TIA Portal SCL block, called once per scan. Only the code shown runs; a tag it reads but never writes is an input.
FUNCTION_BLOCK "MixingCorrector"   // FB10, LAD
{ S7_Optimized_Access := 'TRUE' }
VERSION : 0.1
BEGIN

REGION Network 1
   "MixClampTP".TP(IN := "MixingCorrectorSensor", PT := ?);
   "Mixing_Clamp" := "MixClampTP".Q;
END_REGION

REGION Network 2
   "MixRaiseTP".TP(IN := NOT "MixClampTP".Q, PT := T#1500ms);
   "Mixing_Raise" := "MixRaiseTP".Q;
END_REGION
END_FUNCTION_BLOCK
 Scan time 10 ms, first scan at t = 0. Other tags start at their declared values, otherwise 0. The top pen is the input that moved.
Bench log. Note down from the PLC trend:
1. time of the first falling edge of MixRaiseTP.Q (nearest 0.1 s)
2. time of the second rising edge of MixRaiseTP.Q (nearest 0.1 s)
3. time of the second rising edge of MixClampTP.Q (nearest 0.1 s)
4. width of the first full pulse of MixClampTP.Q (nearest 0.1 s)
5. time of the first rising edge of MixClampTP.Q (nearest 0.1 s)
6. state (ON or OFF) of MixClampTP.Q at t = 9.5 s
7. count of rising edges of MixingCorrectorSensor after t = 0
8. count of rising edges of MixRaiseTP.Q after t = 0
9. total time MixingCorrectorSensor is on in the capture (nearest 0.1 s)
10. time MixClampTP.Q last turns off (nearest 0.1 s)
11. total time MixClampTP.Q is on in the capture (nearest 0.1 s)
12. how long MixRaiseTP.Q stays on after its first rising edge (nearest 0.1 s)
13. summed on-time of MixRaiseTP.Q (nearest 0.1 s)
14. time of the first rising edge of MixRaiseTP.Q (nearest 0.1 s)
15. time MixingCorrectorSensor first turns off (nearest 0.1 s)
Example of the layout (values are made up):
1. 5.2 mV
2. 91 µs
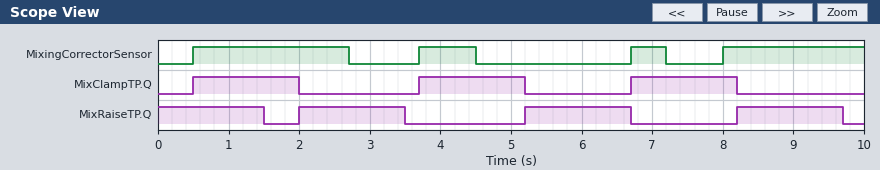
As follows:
1. 1.5 s
2. 5.2 s
3. 3.7 s
4. 1.5 s
5. 0.5 s
6. OFF
7. 4
8. 3
9. 5.5 s
10. 8.2 s
11. 4.5 s
12. 1.5 s
13. 6.0 s
14. 2.0 s
15. 2.7 s
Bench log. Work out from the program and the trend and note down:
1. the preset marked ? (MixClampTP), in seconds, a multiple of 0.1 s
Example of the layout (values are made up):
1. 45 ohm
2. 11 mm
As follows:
1. 1.5 s
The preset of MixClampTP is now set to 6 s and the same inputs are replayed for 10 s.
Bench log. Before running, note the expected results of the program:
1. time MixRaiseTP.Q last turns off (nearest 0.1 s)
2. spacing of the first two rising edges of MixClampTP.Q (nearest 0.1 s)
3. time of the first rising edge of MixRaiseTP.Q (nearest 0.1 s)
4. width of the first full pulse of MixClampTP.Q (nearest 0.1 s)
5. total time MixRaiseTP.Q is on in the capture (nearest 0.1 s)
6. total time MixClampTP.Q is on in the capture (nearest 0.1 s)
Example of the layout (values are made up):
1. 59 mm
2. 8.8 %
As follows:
1. 8.0 s
2. 6.2 s
3. 6.5 s
4. 6.0 s
5. 3.0 s
6. 9.3 s
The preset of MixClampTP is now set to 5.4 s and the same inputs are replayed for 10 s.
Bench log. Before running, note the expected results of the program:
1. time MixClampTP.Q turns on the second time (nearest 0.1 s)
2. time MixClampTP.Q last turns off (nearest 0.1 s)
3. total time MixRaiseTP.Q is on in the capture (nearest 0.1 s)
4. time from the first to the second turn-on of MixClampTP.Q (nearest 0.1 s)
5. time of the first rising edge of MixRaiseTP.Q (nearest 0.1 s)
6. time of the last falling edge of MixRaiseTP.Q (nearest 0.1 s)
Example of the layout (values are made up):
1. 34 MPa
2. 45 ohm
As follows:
1. 6.7 s
2. 5.9 s
3. 3.0 s
4. 6.2 s
5. 5.9 s
6. 7.4 s
